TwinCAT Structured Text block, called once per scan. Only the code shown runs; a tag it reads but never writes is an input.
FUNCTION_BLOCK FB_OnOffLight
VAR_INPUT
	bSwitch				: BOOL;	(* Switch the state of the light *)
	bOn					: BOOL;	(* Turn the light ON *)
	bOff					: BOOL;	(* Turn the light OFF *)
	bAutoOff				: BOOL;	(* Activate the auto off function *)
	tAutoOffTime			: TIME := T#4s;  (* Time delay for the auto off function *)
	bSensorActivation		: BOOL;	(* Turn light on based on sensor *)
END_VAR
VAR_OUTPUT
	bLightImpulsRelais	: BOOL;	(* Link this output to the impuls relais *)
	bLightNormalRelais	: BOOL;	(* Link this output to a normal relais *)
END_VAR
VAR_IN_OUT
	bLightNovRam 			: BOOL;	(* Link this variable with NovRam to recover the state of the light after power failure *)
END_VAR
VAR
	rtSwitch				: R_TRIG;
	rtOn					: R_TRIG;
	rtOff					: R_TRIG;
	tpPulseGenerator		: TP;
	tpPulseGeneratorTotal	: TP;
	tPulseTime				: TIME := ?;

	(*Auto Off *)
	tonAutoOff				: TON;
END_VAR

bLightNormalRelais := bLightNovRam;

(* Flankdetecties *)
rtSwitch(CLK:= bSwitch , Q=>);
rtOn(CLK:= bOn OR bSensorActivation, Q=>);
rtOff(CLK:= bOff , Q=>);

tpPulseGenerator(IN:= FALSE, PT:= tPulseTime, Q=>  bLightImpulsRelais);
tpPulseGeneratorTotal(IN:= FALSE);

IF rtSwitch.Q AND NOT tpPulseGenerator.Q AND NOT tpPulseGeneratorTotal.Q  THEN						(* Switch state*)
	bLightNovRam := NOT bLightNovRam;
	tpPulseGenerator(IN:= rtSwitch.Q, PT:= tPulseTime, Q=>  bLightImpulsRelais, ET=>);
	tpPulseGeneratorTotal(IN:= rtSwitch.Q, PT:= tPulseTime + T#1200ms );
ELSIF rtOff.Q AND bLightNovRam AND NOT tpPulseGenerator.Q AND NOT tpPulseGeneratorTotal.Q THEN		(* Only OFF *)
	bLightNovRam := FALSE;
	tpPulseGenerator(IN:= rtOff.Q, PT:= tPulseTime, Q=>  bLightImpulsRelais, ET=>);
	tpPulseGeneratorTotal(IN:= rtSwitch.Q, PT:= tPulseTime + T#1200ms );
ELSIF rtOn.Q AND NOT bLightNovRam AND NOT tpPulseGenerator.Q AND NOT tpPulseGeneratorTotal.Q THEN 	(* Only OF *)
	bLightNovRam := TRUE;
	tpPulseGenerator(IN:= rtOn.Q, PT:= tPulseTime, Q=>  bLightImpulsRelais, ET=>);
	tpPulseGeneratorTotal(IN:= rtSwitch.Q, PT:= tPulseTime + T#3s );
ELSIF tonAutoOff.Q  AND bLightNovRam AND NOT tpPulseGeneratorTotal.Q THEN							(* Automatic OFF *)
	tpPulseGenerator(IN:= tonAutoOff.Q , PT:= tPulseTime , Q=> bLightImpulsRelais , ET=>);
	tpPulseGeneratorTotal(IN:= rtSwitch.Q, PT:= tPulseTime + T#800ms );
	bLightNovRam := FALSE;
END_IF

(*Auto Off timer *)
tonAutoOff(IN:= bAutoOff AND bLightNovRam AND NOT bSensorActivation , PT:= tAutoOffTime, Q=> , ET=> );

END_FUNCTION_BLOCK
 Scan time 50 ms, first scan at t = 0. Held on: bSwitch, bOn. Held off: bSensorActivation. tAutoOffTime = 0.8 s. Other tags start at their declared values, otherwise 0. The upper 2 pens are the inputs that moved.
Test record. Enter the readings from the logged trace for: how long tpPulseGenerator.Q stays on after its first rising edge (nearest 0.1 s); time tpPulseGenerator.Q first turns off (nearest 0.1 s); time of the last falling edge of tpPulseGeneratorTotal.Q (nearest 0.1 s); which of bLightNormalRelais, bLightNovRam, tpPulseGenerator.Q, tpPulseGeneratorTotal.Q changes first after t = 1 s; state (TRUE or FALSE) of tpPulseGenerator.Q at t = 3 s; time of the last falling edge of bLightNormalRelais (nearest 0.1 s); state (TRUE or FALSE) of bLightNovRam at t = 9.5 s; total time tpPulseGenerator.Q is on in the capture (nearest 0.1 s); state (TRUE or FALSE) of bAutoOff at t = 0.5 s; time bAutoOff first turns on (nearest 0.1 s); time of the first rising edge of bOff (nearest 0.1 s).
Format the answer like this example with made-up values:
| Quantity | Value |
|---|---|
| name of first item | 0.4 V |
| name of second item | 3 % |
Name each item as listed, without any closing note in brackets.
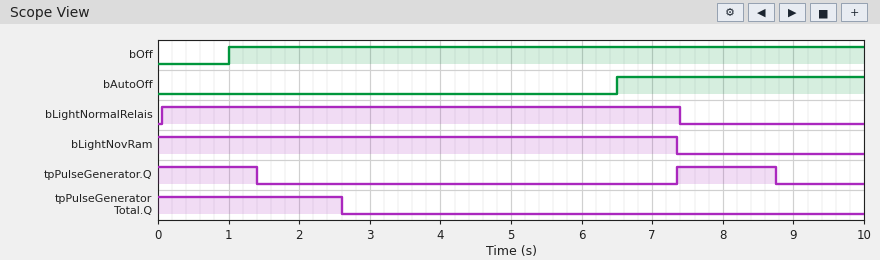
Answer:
| Quantity | Value |
|---|---|
| how long tpPulseGenerator.Q stays on after its first rising edge | 1.4 s |
| time tpPulseGenerator.Q first turns off | 1.4 s |
| time of the last falling edge of tpPulseGeneratorTotal.Q | 2.6 s |
| which of bLightNormalRelais, bLightNovRam, tpPulseGenerator.Q, tpPulseGeneratorTotal.Q changes first after t = 1 s | tpPulseGenerator.Q |
| state (TRUE or FALSE) of tpPulseGenerator.Q at t = 3 s | FALSE |
| time of the last falling edge of bLightNormalRelais | 7.4 s |
| state (TRUE or FALSE) of bLightNovRam at t = 9.5 s | FALSE |
| total time tpPulseGenerator.Q is on in the capture | 2.8 s |
| state (TRUE or FALSE) of bAutoOff at t = 0.5 s | FALSE |
| time bAutoOff first turns on | 6.5 s |
| time of the first rising edge of bOff | 1.0 s |
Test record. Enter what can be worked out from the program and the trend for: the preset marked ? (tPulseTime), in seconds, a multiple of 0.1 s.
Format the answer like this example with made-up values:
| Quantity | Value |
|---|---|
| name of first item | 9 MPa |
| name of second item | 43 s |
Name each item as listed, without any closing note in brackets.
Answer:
| Quantity | Value |
|---|---|
| the preset marked ? (tPulseTime), in seconds, a multiple of 0.1 s | 1.4 s |
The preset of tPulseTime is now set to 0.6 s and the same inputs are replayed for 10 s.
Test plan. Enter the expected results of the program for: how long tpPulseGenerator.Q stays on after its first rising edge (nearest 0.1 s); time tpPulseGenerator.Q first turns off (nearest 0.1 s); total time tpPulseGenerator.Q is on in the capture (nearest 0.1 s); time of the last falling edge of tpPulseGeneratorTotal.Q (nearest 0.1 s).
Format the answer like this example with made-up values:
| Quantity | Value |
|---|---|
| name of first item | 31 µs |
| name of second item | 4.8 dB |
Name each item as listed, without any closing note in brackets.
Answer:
| Quantity | Value |
|---|---|
| how long tpPulseGenerator.Q stays on after its first rising edge | 0.6 s |
| time tpPulseGenerator.Q first turns off | 0.6 s |
| total time tpPulseGenerator.Q is on in the capture | 1.2 s |
| time of the last falling edge of tpPulseGeneratorTotal.Q | 1.8 s |
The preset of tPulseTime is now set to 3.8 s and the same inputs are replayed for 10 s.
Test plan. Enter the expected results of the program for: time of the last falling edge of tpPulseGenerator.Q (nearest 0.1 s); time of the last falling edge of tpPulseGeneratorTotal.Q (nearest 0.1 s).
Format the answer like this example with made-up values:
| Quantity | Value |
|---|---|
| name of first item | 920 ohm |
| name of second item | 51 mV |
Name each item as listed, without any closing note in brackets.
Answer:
| Quantity | Value |
|---|---|
| time of the last falling edge of tpPulseGenerator.Q | 3.8 s |
| time of the last falling edge of tpPulseGeneratorTotal.Q | 5.0 s |
